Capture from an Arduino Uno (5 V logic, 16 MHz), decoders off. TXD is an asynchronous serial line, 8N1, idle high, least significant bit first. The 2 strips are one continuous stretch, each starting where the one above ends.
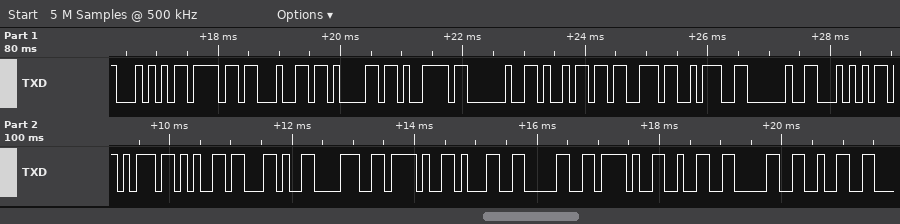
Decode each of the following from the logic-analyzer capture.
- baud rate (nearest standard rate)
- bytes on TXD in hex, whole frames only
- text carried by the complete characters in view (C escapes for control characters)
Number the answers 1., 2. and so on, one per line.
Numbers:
1. 9600 baud
2. 54 6F 64 61 79 20 69 73 3A 20 54 75 65 2C 38 2F 31 30 2F 32 30 32
3. "Today is: Tue,8/10/202"
